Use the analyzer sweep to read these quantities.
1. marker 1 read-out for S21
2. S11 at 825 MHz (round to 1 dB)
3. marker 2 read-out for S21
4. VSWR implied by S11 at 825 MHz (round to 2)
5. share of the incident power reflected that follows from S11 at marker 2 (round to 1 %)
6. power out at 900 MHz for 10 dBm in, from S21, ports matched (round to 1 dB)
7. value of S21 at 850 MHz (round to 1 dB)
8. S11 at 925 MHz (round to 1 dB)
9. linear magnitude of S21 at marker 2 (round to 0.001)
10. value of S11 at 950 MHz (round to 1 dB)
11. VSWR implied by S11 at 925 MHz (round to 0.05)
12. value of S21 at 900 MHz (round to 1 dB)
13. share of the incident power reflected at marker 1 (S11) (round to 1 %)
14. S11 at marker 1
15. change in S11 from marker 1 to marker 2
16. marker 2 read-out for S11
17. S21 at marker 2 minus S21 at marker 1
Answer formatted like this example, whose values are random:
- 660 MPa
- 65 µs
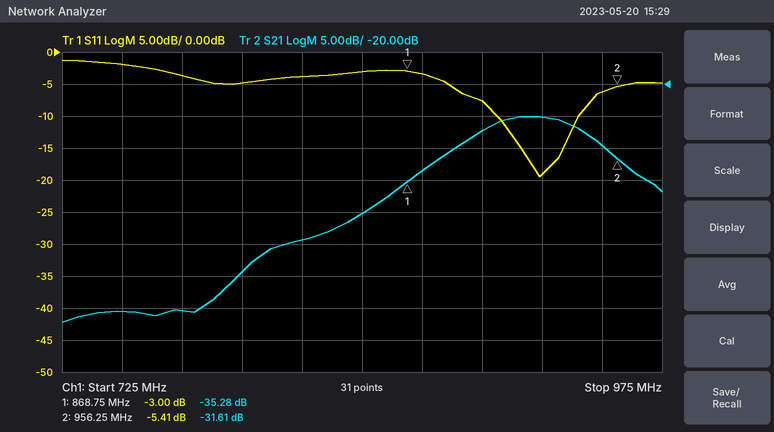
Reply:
- -35.28 dB
- -4 dB
- -31.61 dB
- 4
- 29 %
- -17 dBm
- -40 dB
- -19 dB
- 0.026
- -6 dB
- 1.25
- -27 dB
- 50 %
- -3.00 dB
- -2.41 dB
- -5.41 dB
- 3.67 dB
